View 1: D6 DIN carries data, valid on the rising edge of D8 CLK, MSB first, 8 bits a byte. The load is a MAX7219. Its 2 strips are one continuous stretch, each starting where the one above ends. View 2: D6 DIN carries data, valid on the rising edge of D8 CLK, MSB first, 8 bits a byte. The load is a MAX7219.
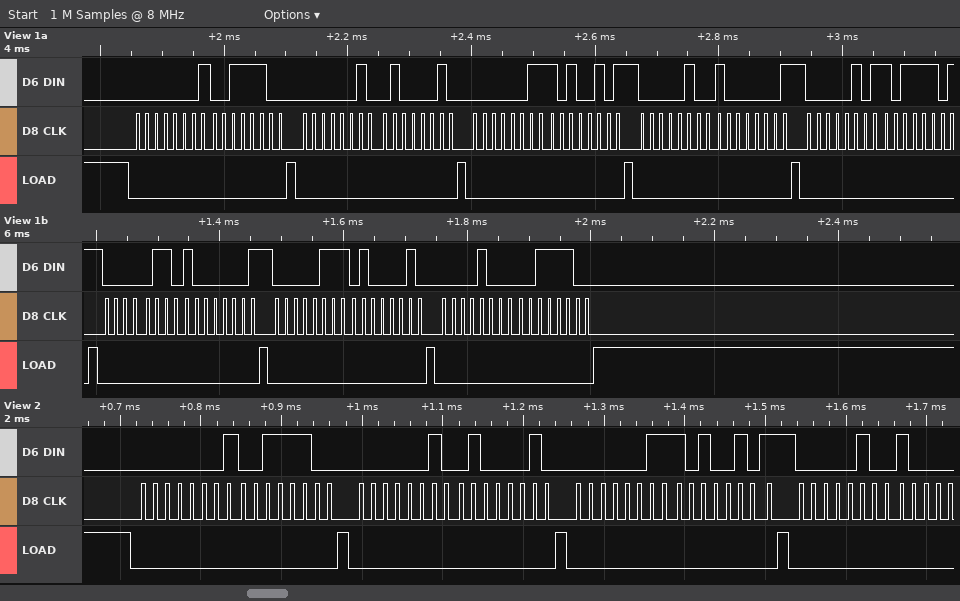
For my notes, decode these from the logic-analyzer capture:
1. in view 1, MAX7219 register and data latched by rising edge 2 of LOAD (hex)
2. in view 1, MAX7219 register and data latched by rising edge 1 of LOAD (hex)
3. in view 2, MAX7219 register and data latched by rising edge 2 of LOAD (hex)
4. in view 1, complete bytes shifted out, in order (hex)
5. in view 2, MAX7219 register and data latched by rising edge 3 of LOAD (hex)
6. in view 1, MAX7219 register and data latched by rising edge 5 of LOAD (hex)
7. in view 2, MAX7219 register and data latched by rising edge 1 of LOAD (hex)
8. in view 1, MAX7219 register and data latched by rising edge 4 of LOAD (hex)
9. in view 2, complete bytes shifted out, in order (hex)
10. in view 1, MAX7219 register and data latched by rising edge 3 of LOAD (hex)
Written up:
register 0x2, data 0x42
register 0x1, data 0x3C
register 0x2, data 0x42
01 3C 02 42 03 A5 04 81 05 BD 06 81 07 42 08 3C
register 0x3, data 0xA5
register 0x5, data 0xBD
register 0x1, data 0x3C
register 0x4, data 0x81
01 3C 02 42 03 A5 04
register 0x3, data 0xA5
